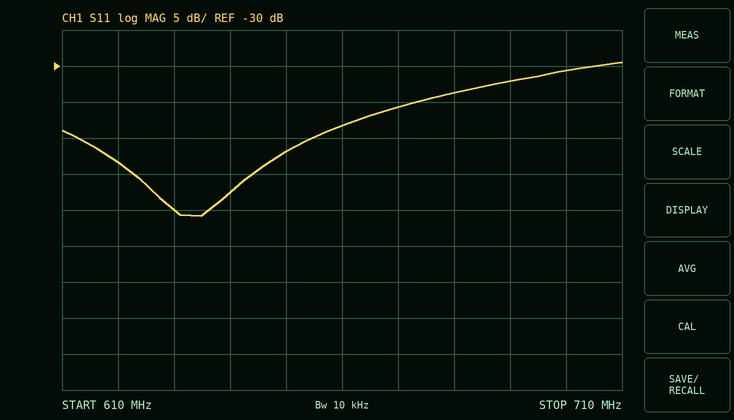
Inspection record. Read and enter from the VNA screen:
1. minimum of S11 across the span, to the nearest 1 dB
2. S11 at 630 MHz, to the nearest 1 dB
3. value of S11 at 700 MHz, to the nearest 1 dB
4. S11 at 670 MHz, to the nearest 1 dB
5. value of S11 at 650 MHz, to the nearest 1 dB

-51 dB
-50 dB
-31 dB
-36 dB
-42 dB
